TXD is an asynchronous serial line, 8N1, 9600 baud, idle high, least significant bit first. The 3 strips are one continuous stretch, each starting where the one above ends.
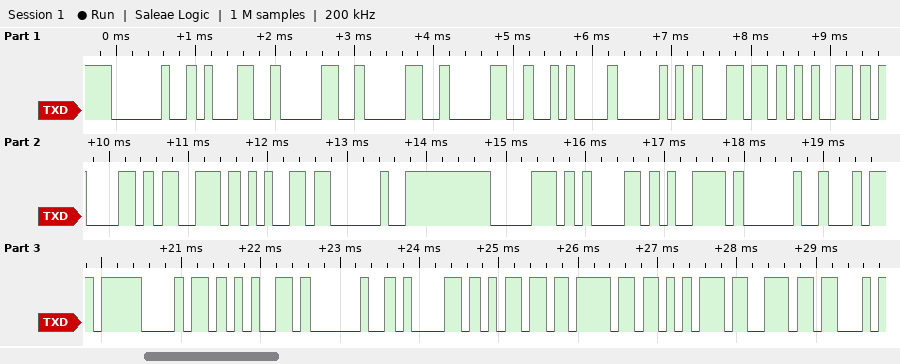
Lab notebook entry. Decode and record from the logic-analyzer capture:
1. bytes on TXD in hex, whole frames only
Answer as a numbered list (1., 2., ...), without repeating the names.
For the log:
1. 20 31 30 30 30 0A 50 6C 65 61 73 65 20 70 61 79 20 74 68 65 20 61 6D 6F 75 6E
